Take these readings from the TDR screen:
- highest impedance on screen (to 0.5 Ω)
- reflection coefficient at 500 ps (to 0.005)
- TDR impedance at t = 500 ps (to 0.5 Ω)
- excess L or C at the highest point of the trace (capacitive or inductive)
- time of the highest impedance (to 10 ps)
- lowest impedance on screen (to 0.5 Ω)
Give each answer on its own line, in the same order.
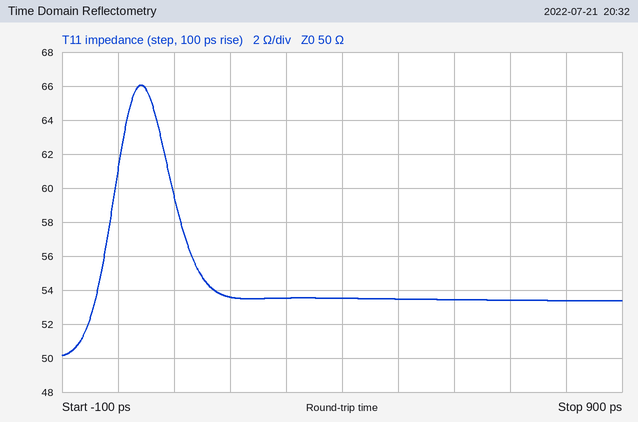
66.0 Ω
+0.035
53.5 Ω
inductive
40 ps
50.0 Ω
